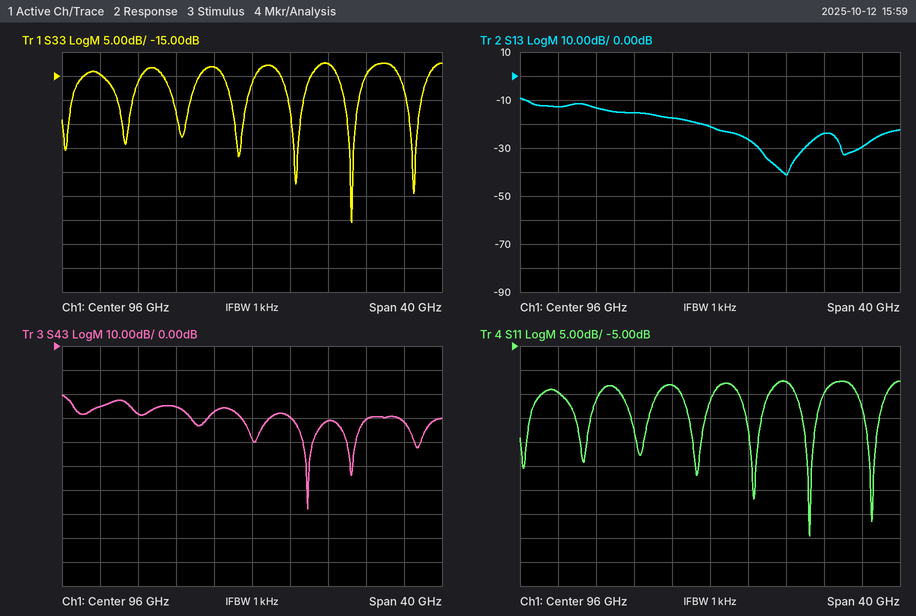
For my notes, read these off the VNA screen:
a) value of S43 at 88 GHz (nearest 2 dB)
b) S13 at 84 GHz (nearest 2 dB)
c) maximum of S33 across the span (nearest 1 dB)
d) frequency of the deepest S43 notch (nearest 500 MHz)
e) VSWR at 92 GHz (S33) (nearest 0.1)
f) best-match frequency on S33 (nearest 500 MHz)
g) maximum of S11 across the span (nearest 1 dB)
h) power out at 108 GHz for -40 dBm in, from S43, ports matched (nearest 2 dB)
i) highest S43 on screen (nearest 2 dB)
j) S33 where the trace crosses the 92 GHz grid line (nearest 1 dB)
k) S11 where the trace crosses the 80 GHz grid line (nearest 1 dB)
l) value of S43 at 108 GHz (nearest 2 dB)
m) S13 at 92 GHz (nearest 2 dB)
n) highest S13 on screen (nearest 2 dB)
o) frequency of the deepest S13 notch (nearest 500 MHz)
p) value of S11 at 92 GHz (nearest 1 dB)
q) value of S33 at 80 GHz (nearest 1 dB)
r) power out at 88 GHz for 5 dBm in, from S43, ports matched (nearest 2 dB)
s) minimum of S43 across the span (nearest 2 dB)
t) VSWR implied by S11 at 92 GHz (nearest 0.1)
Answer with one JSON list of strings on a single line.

["-26 dB", "-14 dB", "-12 dB", "102.0 GHz", "1.6", "106.5 GHz", "-12 dB", "-70 dBm", "-20 dB", "-13 dB", "-15 dB", "-30 dB", "-18 dB", "-10 dB", "104.0 GHz", "-13 dB", "-15 dB", "-20 dBm", "-68 dB", "1.6"]
